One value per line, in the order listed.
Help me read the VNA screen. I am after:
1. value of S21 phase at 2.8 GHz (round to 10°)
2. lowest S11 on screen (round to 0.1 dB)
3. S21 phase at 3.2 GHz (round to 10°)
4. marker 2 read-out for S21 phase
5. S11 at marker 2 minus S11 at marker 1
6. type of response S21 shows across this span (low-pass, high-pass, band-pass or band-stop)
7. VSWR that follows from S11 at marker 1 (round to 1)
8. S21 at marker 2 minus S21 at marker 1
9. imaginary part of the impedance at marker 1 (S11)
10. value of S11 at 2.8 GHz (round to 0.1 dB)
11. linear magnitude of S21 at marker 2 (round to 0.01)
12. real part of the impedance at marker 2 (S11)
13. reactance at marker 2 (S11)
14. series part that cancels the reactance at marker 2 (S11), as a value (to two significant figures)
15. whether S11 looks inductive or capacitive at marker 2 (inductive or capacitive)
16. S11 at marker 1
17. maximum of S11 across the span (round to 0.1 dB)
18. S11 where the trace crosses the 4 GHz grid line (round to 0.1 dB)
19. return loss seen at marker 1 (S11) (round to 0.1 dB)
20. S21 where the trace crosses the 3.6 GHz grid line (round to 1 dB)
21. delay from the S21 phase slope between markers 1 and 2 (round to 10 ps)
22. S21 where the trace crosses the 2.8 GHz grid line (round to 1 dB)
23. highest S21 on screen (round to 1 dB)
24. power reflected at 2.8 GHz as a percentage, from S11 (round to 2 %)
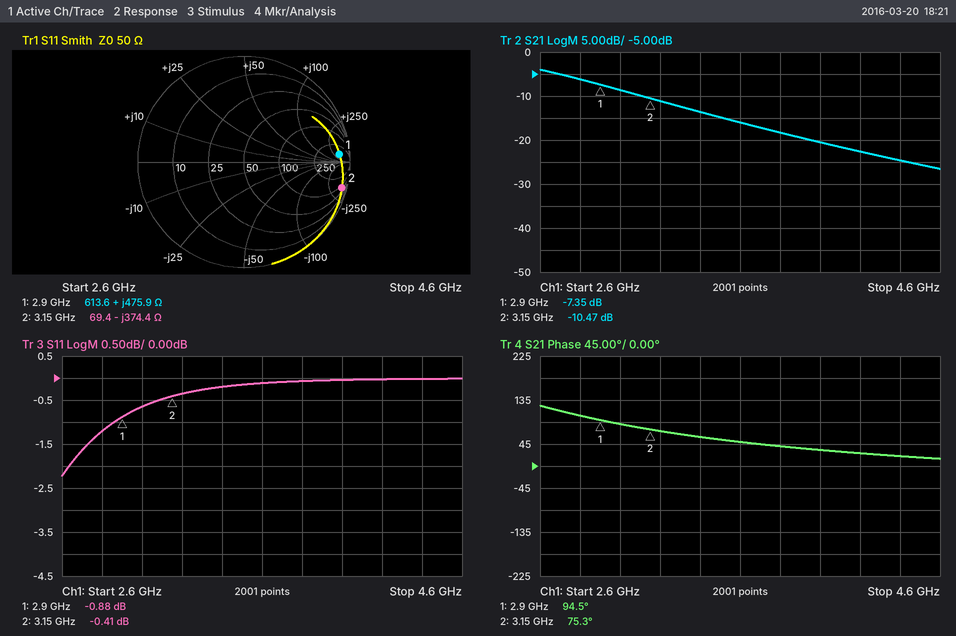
100°
-2.2 dB
70°
75.3°
0.47 dB
low-pass
20
-3.12 dB
+475.9 Ω
-1.2 dB
0.30
69.4 Ω
-374.4 Ω
19 nH
capacitive
-0.88 dB
0.0 dB
0.0 dB
0.9 dB
-16 dB
210 ps
-6 dB
-4 dB
76 %
